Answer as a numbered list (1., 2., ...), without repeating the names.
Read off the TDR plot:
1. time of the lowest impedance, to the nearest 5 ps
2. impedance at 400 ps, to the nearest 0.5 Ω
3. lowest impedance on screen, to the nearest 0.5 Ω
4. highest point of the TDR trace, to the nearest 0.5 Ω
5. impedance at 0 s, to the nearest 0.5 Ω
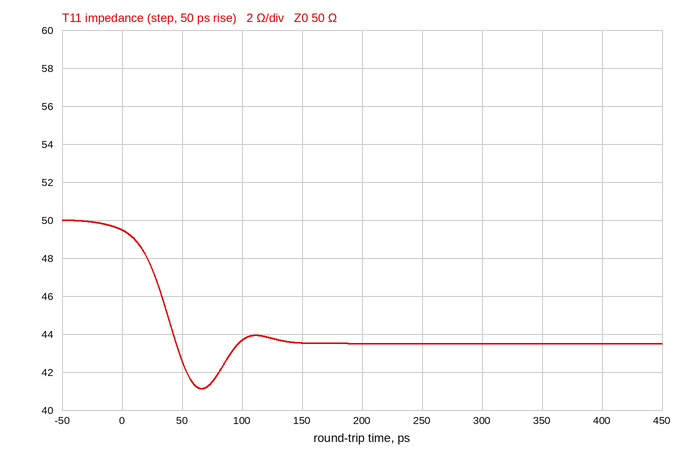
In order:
1. 65 ps
2. 43.5 Ω
3. 41.0 Ω
4. 50.0 Ω
5. 49.5 Ω
